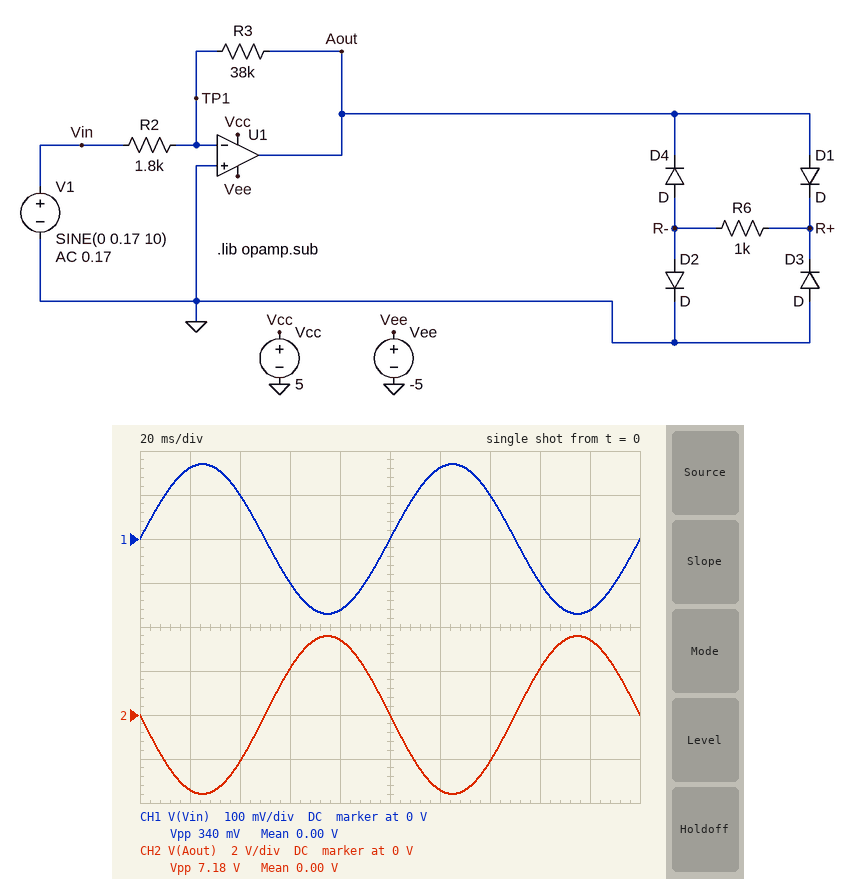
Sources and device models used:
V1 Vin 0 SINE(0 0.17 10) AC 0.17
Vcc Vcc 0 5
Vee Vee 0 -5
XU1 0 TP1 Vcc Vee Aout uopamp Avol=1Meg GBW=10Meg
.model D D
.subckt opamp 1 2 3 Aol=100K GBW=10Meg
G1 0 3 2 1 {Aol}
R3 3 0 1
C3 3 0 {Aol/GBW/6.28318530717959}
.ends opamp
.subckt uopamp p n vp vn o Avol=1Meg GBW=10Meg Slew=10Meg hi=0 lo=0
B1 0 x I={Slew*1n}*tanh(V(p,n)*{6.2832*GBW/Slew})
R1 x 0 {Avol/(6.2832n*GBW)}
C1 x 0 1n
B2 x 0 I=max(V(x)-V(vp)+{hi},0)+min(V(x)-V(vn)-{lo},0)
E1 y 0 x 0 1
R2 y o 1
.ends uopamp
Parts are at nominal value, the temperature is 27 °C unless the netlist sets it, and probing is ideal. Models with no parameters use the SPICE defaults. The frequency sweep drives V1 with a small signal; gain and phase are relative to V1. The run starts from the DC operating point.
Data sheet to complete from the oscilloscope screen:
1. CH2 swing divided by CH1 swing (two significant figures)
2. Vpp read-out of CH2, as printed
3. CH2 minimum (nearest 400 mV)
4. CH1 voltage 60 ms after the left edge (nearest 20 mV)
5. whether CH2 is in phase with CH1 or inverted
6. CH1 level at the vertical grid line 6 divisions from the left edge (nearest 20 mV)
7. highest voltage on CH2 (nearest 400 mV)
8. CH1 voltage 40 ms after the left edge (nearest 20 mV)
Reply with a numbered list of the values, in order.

1. 21
2. 7.18 V
3. -3.6 V
4. -100 mV
5. inverted
6. 160 mV
7. 3.6 V
8. 100 mV
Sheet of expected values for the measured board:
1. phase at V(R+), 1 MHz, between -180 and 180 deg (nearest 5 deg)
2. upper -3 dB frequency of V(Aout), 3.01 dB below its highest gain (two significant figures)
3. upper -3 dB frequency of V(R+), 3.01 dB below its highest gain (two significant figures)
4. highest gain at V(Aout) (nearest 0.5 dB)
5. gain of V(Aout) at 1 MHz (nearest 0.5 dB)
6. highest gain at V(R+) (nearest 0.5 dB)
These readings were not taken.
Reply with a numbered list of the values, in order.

1. 115 deg
2. 450 kHz
3. 450 kHz
4. 26.5 dB
5. 19.0 dB
6. 20.5 dB
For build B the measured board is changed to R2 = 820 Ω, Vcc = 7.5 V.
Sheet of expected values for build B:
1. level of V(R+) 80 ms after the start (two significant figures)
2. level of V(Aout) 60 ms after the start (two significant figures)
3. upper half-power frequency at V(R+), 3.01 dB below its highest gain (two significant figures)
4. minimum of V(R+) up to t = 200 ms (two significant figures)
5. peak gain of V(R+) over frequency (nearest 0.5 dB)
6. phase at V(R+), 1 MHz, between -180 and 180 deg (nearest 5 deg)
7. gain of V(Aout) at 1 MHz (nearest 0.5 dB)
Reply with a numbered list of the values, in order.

1. 6.8 V
2. 4.6 V
3. 210 kHz
4. -690 mV
5. 27.5 dB
6. 100 deg
7. 19.5 dB
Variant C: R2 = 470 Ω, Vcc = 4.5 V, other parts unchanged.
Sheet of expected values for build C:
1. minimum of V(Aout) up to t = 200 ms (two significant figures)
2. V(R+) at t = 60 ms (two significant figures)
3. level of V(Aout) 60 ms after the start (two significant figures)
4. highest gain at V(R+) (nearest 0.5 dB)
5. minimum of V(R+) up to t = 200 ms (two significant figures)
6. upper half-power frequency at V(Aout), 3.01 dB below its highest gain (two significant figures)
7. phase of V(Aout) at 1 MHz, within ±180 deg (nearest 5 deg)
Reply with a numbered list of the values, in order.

1. -5.0 V
2. 3.8 V
3. 4.5 V
4. 32.0 dB
5. -690 mV
6. 120 kHz
7. 95 deg
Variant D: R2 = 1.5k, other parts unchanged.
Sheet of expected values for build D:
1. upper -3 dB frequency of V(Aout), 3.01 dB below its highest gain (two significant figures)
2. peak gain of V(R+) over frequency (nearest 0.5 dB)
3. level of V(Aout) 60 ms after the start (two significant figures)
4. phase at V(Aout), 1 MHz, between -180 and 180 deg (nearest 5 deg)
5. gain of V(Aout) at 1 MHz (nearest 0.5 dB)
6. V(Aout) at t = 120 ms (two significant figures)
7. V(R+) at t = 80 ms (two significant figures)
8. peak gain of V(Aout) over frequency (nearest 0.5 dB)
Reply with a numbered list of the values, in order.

1. 380 kHz
2. 22.0 dB
3. 2.5 V
4. 110 deg
5. 19.0 dB
6. -4.1 V
7. 3.4 V
8. 28.0 dB
